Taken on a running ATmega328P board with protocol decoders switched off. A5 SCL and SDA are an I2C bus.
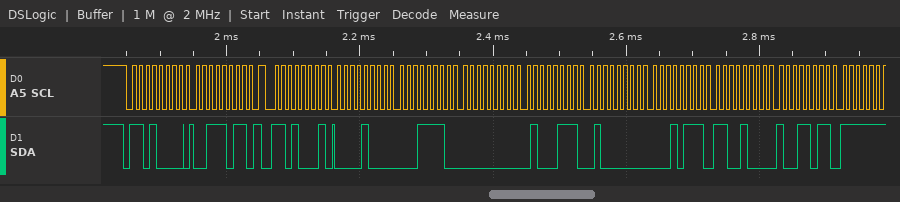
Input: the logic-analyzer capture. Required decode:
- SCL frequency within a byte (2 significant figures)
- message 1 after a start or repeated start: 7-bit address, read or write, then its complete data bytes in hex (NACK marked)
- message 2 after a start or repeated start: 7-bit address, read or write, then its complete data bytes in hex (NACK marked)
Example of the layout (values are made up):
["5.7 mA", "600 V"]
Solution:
["100 kHz", "0x68 write: 3B", "0x68 read: 08 1E 00 47 40 17 C8 9B"]
